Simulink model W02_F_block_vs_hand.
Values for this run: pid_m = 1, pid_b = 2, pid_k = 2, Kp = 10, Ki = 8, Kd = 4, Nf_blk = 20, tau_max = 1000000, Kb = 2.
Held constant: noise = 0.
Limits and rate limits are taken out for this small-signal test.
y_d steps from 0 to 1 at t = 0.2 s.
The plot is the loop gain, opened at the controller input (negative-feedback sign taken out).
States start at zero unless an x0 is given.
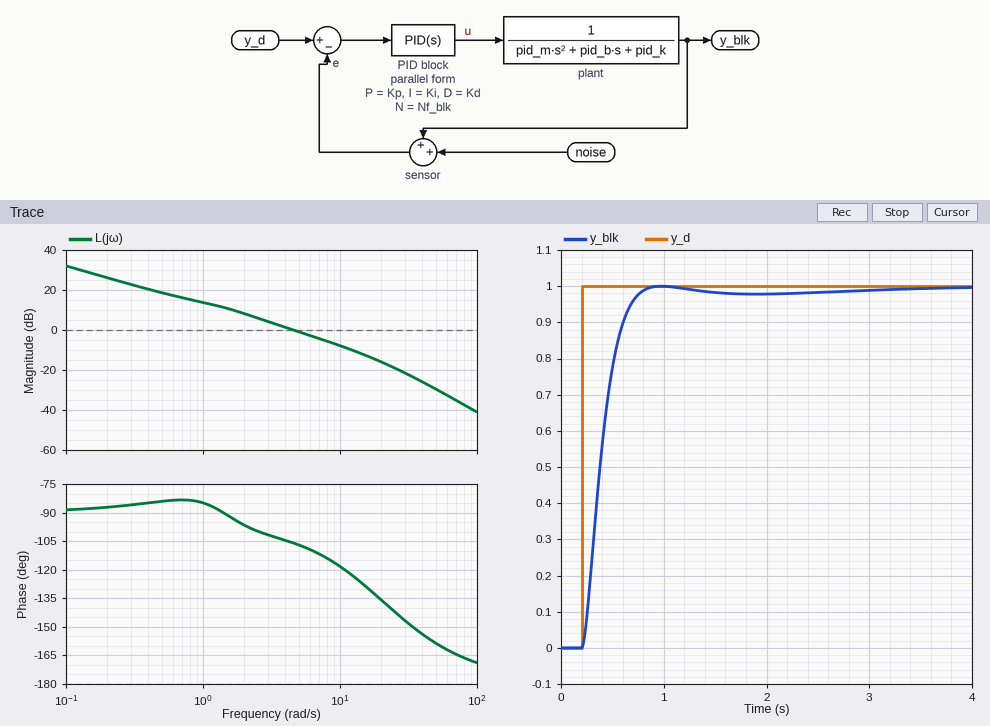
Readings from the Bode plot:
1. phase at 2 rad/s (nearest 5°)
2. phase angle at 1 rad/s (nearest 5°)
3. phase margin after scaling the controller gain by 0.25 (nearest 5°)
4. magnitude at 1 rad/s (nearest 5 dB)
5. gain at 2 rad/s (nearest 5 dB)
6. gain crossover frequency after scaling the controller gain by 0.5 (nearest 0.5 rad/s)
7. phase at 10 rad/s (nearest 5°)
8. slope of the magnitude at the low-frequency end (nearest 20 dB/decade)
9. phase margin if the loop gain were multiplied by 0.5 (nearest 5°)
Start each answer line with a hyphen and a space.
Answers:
- -95°
- -85°
- 90°
- 15 dB
- 10 dB
- 2.5 rad/s
- -120°
- -20 dB/decade
- 80°
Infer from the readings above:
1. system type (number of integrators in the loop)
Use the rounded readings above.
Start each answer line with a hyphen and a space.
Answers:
- 1
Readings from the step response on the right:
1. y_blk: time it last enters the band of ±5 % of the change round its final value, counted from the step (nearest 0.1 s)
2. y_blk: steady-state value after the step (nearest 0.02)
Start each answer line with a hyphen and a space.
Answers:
- 0.5 s
- 1.00
